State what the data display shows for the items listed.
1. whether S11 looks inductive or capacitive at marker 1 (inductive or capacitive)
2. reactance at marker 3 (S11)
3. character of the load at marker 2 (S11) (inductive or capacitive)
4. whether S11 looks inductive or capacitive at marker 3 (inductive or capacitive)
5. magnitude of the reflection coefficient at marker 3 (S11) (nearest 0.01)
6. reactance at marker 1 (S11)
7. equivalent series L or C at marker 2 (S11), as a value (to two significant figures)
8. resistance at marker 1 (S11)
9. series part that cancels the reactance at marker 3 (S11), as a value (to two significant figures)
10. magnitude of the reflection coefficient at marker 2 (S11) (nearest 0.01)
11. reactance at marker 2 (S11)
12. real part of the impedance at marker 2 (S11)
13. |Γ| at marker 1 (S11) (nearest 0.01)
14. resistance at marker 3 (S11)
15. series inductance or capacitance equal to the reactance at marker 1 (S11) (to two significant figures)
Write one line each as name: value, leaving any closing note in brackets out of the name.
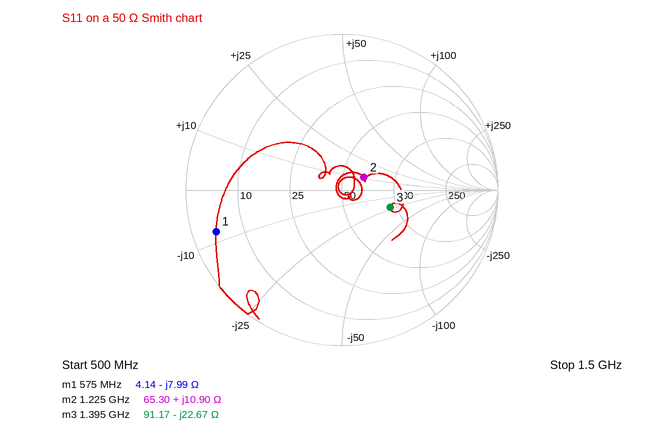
whether S11 looks inductive or capacitive at marker 1: capacitive
reactance at marker 3: -22.67 Ω
character of the load at marker 2 (S11): inductive
whether S11 looks inductive or capacitive at marker 3: capacitive
magnitude of the reflection coefficient at marker 3 (S11): 0.33
reactance at marker 1: -7.99 Ω
equivalent series L or C at marker 2 (S11), as a value: 1.4 nH
resistance at marker 1: 4.14 Ω
series part that cancels the reactance at marker 3 (S11), as a value: 2.6 nH
magnitude of the reflection coefficient at marker 2 (S11): 0.16
reactance at marker 2: +10.90 Ω
real part of the impedance at marker 2: 65.30 Ω
|Γ| at marker 1 (S11): 0.85
resistance at marker 3: 91.17 Ω
series inductance or capacitance equal to the reactance at marker 1 (S11): 35 pF
